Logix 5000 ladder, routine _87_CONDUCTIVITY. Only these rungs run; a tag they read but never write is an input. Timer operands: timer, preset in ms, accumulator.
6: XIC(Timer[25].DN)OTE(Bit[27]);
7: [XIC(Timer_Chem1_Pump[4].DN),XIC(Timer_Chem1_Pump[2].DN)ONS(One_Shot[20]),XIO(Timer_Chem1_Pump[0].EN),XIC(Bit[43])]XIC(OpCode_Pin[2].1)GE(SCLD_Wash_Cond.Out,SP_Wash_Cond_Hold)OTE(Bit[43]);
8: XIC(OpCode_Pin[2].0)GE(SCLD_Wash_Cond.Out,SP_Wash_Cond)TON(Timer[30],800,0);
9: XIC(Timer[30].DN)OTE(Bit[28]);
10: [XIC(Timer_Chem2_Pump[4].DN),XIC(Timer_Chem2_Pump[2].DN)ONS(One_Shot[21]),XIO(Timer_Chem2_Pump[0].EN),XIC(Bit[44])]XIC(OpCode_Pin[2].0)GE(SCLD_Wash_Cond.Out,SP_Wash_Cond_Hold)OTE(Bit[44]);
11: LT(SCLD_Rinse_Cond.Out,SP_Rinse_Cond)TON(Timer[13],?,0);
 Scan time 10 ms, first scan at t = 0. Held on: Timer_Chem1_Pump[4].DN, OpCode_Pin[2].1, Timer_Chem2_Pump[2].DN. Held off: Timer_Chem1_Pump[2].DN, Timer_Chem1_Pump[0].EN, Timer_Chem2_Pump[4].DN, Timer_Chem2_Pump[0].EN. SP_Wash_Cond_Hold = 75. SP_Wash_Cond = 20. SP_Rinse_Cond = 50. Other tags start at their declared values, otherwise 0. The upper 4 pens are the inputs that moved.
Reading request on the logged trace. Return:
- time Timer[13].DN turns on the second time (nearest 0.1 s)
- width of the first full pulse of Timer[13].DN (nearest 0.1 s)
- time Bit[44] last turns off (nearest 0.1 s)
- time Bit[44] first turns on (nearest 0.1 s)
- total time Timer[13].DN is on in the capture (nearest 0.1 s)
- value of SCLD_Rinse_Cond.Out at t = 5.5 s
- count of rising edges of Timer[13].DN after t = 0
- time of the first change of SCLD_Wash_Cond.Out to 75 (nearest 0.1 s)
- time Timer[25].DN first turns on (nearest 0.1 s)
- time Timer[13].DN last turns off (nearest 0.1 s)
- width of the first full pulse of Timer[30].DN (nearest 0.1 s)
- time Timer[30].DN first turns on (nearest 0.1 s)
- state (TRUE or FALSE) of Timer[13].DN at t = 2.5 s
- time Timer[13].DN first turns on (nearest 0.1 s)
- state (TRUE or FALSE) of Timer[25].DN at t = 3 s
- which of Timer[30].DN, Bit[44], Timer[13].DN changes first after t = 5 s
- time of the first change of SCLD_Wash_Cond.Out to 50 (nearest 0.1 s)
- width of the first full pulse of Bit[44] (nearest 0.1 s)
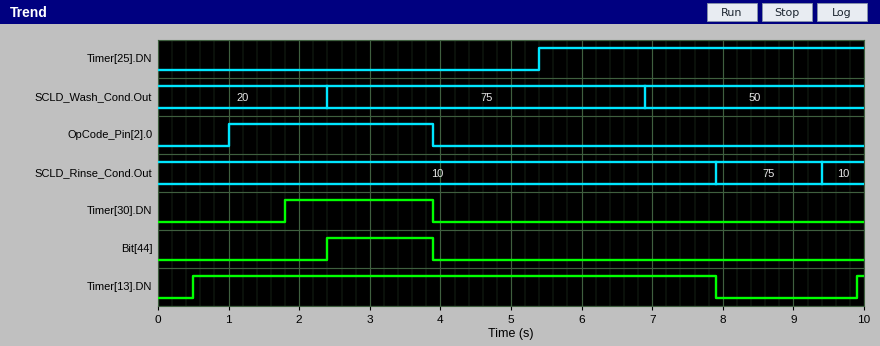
9.9 s
7.4 s
3.9 s
2.4 s
7.5 s
10
2
2.4 s
5.4 s
7.9 s
2.1 s
1.8 s
TRUE
0.5 s
FALSE
Timer[13].DN
6.9 s
1.5 s
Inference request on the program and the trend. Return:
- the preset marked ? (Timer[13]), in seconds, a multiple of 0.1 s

0.5 s
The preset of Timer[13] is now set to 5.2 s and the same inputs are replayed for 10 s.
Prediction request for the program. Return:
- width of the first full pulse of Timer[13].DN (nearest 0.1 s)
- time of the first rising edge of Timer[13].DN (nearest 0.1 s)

2.7 s
5.2 s
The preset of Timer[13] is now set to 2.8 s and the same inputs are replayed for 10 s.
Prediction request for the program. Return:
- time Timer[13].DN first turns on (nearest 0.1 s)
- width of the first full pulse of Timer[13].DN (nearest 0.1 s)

2.8 s
5.1 s
